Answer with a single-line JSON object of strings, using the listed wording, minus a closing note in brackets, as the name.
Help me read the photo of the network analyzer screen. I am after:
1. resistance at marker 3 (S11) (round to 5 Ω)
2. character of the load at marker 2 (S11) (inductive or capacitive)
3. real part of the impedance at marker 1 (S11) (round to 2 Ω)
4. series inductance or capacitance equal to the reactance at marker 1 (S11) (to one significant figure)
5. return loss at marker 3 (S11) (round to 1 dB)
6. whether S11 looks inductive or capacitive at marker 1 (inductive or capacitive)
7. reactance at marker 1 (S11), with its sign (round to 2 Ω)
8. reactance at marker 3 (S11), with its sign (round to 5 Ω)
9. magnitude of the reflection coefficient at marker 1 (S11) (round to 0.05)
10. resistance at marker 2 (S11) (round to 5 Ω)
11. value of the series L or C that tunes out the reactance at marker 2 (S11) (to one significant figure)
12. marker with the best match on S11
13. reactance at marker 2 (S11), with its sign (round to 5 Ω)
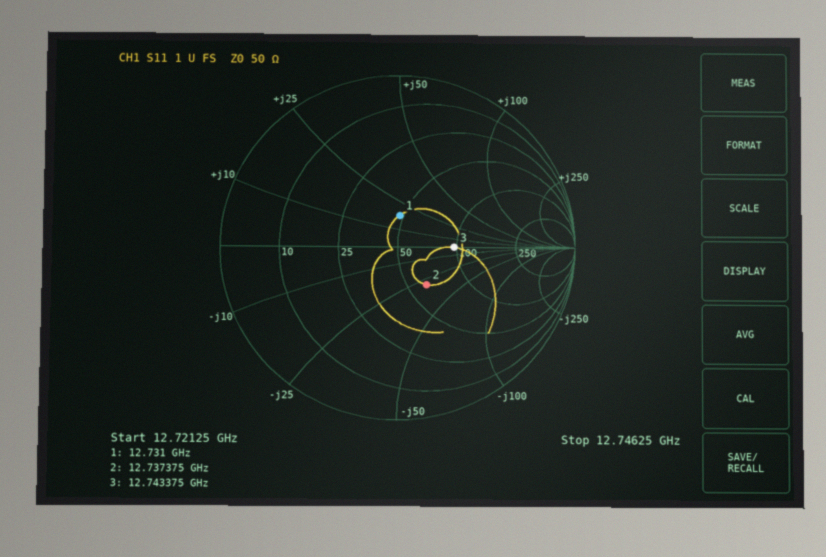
{"resistance at marker 3 (S11)": "95 Ω", "character of the load at marker 2 (S11)": "capacitive", "real part of the impedance at marker 1 (S11)": "48 Ω", "series inductance or capacitance equal to the reactance at marker 1 (S11)": "200 pH", "return loss at marker 3 (S11)": "10 dB", "whether S11 looks inductive or capacitive at marker 1": "inductive", "reactance at marker 1 (S11), with its sign": "+18 Ω", "reactance at marker 3 (S11), with its sign": "0 Ω", "magnitude of the reflection coefficient at marker 1 (S11)": "0.20", "resistance at marker 2 (S11)": "60 Ω", "value of the series L or C that tunes out the reactance at marker 2 (S11)": "400 pH", "marker with the best match on S11": "marker 1", "reactance at marker 2 (S11), with its sign": "-30 Ω"}
